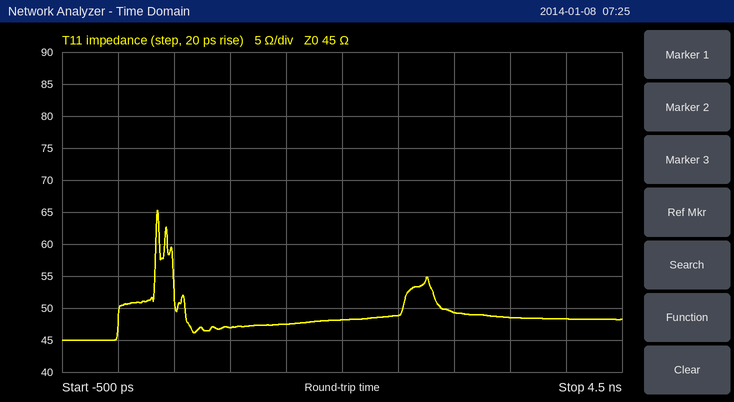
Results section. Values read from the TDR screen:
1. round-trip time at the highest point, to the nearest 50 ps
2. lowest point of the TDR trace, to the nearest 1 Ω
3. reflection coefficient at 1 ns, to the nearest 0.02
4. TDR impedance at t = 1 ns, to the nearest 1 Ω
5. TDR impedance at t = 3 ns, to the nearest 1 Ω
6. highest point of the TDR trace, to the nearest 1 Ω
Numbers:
350 ps
45 Ω
+0.02
47 Ω
49 Ω
65 Ω
